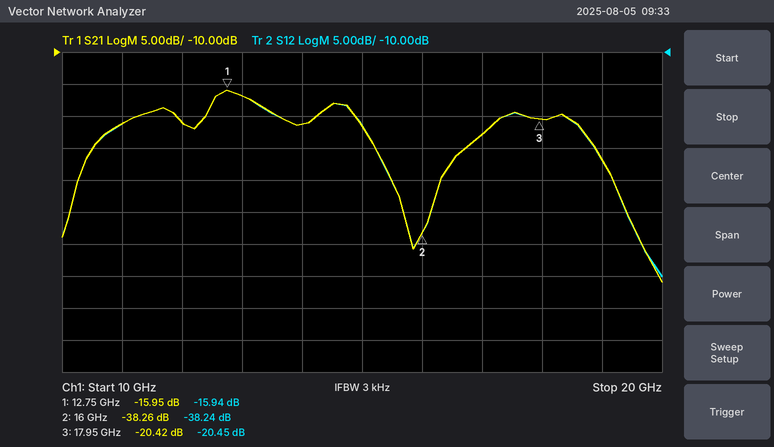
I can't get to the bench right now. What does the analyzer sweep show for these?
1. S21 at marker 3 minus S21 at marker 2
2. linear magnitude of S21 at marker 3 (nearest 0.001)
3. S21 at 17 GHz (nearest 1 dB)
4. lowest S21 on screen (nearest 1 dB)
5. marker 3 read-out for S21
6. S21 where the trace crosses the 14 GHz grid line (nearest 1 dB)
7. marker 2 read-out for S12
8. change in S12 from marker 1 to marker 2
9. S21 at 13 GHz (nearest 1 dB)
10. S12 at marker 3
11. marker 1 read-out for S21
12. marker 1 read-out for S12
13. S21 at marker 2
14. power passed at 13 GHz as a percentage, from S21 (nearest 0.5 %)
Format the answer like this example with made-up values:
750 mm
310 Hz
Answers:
17.84 dB
0.095
-23 dB
-46 dB
-20.42 dB
-21 dB
-38.24 dB
-22.30 dB
-17 dB
-20.45 dB
-15.95 dB
-15.94 dB
-38.26 dB
2.0 %
